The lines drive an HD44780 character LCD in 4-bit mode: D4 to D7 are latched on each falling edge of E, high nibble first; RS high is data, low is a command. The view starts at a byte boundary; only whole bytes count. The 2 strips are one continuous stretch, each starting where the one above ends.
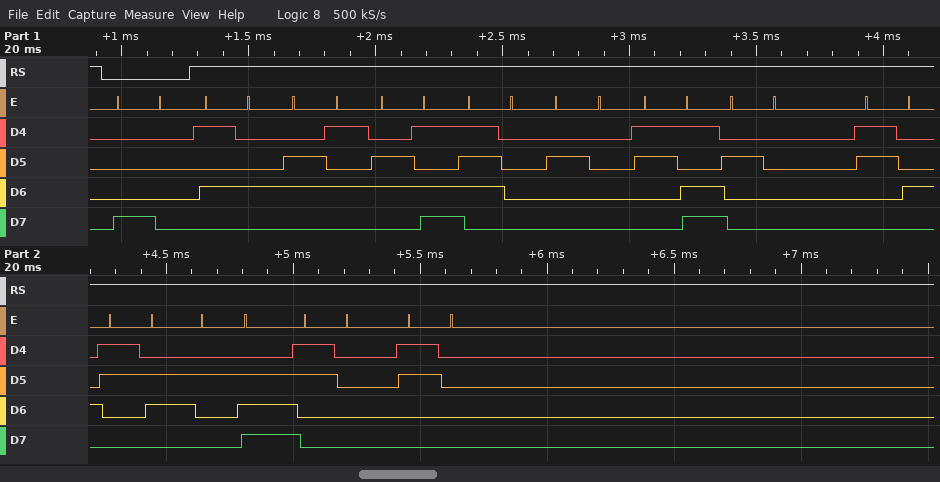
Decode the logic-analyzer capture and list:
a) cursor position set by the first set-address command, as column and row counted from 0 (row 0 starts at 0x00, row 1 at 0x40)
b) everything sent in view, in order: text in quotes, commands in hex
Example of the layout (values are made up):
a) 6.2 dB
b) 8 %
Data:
a) column 0, row 0
b) 0x80 "Temp = 46.00"
